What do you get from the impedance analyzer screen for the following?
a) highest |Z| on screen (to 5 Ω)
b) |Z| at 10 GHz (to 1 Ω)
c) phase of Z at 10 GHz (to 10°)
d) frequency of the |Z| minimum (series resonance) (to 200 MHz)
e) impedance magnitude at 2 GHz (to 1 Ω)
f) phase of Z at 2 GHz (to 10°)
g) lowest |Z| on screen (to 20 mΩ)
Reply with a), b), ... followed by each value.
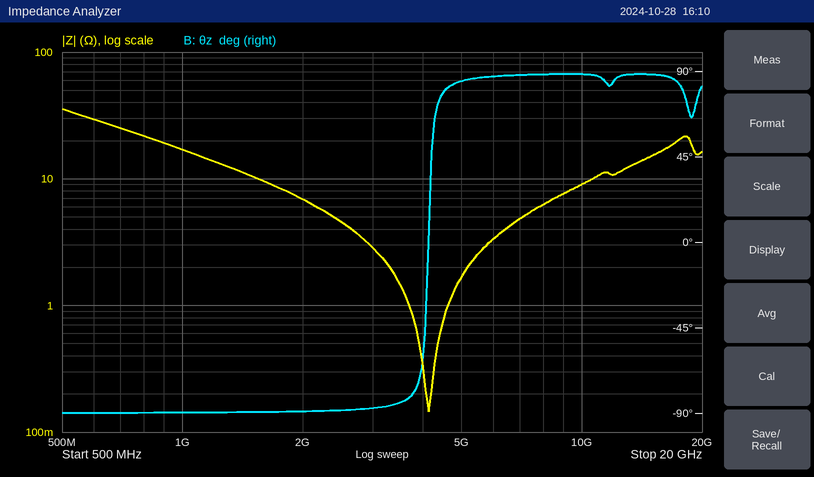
a) 35 Ω
b) 9 Ω
c) 90°
d) 4.2 GHz
e) 7 Ω
f) -90°
g) 140 mΩ
